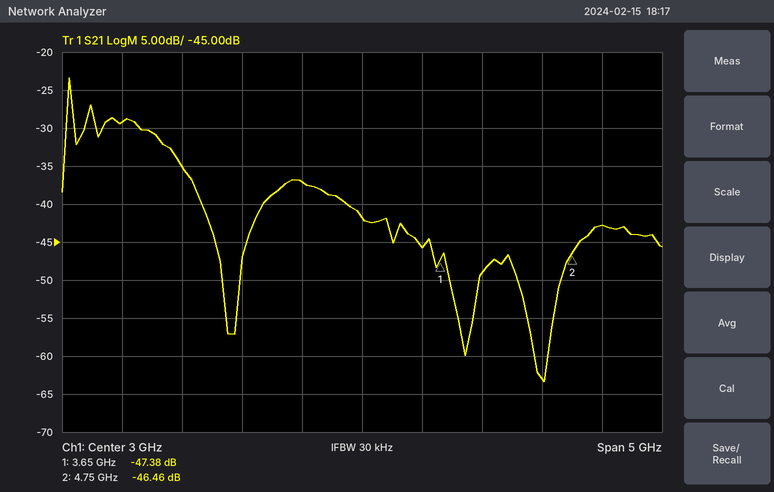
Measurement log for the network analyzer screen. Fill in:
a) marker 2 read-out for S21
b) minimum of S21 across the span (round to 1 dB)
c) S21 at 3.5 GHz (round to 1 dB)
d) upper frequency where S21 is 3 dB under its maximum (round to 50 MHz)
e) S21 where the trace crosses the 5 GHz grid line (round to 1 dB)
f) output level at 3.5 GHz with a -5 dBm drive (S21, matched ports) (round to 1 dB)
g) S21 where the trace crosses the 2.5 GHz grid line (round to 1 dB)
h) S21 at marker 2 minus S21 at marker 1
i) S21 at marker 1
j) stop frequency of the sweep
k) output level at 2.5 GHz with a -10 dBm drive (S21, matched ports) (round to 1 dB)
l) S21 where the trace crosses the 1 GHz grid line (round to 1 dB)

-46.46 dB
-63 dB
-46 dB
600 MHz
-43 dB
-51 dBm
-37 dB
0.92 dB
-47.38 dB
5.5 GHz
-47 dBm
-29 dB
